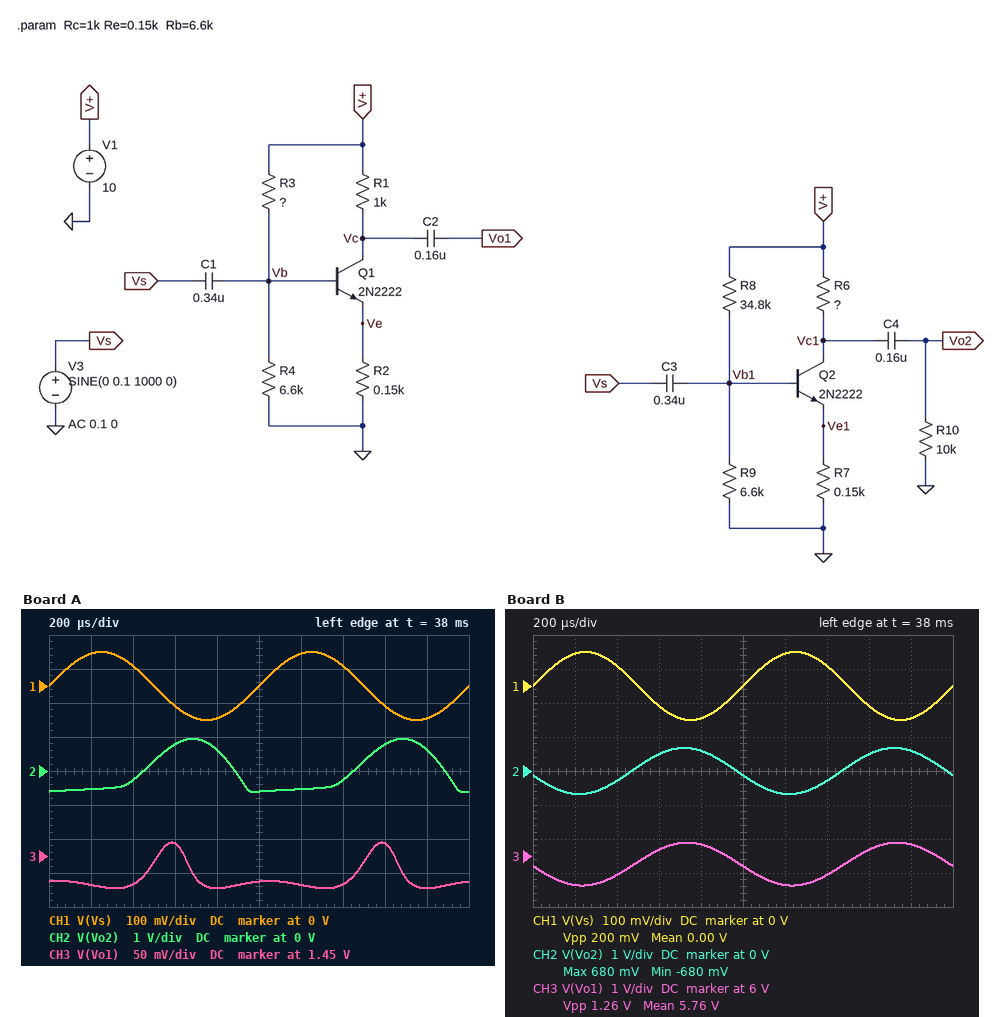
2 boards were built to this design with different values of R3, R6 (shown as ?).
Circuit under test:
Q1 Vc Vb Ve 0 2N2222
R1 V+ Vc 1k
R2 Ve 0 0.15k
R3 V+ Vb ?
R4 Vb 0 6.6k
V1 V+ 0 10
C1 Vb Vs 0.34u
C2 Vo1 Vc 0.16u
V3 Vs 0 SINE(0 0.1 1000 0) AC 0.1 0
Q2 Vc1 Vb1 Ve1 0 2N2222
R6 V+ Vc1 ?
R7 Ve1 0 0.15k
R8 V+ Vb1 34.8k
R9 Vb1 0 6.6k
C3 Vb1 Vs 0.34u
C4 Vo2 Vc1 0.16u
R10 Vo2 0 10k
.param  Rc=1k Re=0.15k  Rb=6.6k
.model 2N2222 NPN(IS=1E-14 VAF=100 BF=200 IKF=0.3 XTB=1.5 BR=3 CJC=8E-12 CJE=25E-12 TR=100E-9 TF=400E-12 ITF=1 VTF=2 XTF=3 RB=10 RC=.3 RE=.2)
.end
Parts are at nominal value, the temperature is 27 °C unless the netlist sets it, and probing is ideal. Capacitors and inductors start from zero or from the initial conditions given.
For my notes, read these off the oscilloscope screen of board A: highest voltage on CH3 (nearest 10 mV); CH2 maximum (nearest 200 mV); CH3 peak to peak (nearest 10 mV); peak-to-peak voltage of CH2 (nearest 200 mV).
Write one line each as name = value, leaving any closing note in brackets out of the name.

highest voltage on CH3 = 1.47 V
CH2 maximum = 1.0 V
CH3 peak to peak = 70 mV
peak-to-peak voltage of CH2 = 1.6 V
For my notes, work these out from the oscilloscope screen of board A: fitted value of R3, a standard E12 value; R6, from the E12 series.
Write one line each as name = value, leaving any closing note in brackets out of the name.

fitted value of R3, a standard E12 value = 15 kΩ
R6, from the E12 series = 2.7 kΩ
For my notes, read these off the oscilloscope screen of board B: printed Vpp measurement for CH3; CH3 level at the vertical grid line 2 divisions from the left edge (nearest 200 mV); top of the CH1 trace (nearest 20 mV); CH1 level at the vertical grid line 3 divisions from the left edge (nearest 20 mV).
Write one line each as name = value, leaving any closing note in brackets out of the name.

printed Vpp measurement for CH3 = 1.26 V
CH3 level at the vertical grid line 2 divisions from the left edge = 5.4 V
top of the CH1 trace = 100 mV
CH1 level at the vertical grid line 3 divisions from the left edge = -60 mV
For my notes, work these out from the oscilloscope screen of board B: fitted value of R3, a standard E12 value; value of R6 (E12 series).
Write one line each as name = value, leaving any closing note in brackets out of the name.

fitted value of R3, a standard E12 value = 39 kΩ
value of R6 = 1.2 kΩ
